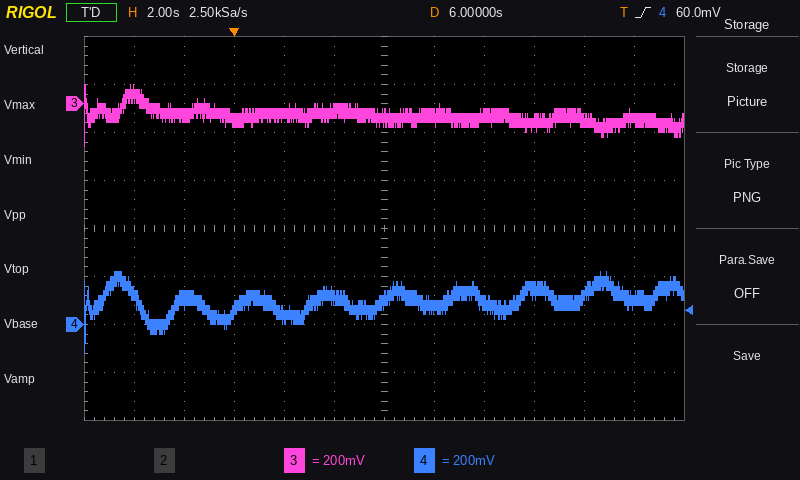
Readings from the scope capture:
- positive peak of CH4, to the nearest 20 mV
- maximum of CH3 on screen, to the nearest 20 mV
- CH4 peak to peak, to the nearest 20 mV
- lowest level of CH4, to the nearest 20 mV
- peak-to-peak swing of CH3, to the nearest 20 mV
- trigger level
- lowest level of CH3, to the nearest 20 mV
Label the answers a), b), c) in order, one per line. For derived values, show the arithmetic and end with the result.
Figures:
a) 220 mV
b) 80 mV
c) 220 mV − (-120 mV) = 340 mV
d) -120 mV
e) 80 mV − (-180 mV) = 260 mV
f) 60.0 mV
g) -180 mV
